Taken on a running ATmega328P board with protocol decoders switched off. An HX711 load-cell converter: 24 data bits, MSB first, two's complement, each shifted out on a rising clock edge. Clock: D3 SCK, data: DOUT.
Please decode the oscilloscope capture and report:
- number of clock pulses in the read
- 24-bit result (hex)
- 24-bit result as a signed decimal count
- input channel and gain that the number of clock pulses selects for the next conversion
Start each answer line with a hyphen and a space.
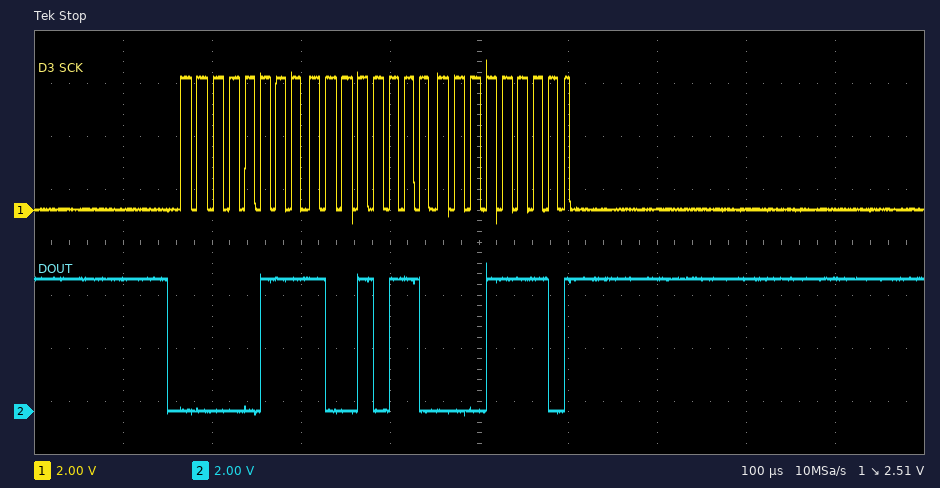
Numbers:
- 25
- 0x07961E
- 497182
- channel A, gain 128
